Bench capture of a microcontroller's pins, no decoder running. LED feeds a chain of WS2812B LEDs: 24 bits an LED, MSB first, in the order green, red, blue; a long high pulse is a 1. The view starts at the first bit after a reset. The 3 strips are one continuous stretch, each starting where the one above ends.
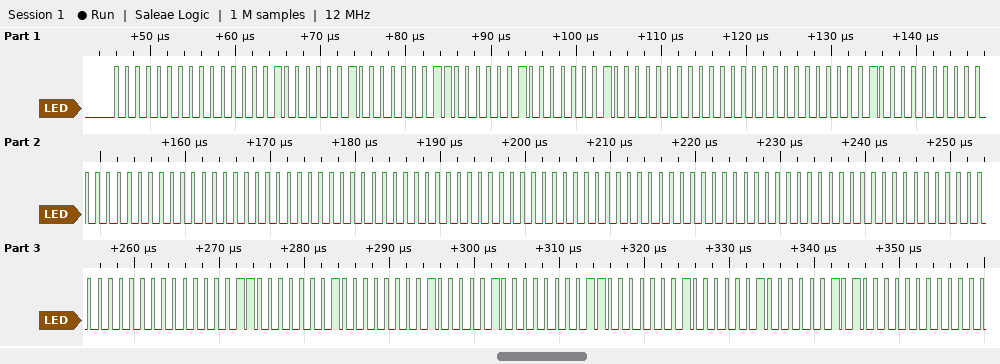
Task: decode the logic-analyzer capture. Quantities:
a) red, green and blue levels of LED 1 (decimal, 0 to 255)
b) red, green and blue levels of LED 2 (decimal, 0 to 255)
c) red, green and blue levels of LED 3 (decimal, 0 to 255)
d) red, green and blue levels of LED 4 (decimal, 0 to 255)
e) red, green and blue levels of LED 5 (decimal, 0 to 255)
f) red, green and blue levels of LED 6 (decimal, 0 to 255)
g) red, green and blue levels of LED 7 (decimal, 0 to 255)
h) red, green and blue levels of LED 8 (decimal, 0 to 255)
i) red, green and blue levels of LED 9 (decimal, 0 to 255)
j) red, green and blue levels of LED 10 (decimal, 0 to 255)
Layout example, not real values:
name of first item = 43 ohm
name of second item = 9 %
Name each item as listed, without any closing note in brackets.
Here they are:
red, green and blue levels of LED 1 = 1, 0, 2
red, green and blue levels of LED 2 = 2, 3, 2
red, green and blue levels of LED 3 = 0, 0, 1
red, green and blue levels of LED 4 = 0, 0, 0
red, green and blue levels of LED 5 = 0, 0, 0
red, green and blue levels of LED 6 = 0, 0, 0
red, green and blue levels of LED 7 = 0, 0, 0
red, green and blue levels of LED 8 = 6, 0, 2
red, green and blue levels of LED 9 = 4, 1, 3
red, green and blue levels of LED 10 = 2, 1, 5
